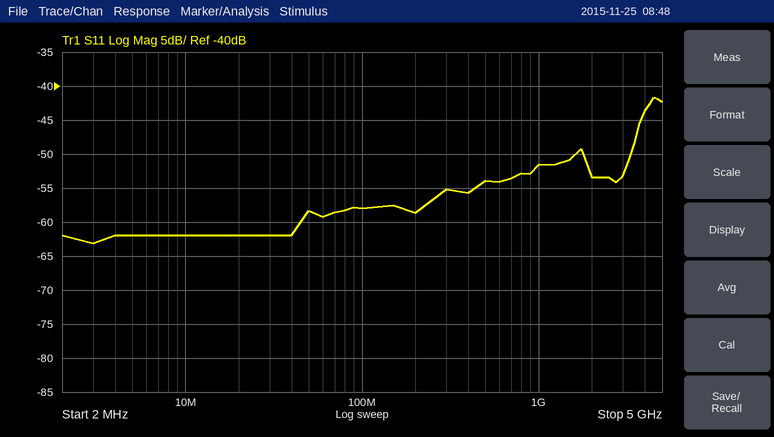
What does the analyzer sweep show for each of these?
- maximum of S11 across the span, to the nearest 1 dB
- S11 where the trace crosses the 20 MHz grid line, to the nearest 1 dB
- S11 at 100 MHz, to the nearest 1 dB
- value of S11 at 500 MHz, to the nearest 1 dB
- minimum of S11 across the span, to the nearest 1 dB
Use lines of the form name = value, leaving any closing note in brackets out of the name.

maximum of S11 across the span, to the nearest 1 dB = -42 dB
S11 where the trace crosses the 20 MHz grid line, to the nearest 1 dB = -62 dB
S11 at 100 MHz, to the nearest 1 dB = -58 dB
value of S11 at 500 MHz, to the nearest 1 dB = -54 dB
minimum of S11 across the span, to the nearest 1 dB = -63 dB
